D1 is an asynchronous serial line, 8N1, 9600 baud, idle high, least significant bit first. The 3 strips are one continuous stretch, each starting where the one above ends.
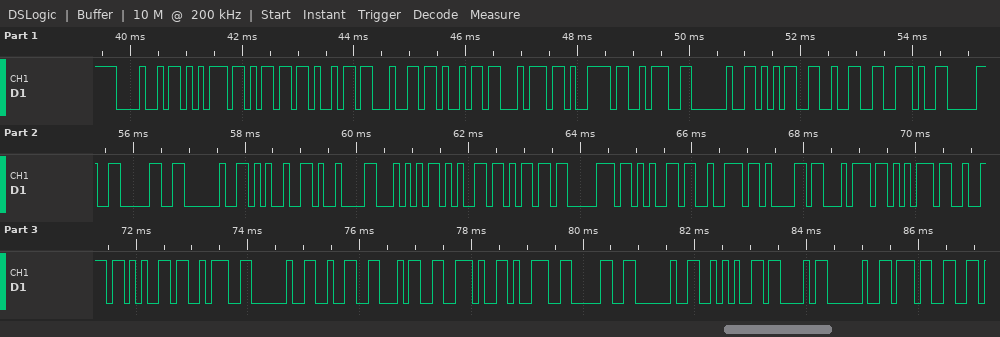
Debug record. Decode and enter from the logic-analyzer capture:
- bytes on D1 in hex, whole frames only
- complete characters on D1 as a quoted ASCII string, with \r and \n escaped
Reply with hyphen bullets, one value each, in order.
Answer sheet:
- 48 75 6D 69 64 69 74 79 3A 20 35 32 2E 30 30 20 25 09 54 65 6D 70 65 72 61 74 75 72 65 3A 20 32 34 2E 39 30 20 2A 43 20 37
- "Humidity: 52.00 %\tTemperature: 24.90 *C 7"
